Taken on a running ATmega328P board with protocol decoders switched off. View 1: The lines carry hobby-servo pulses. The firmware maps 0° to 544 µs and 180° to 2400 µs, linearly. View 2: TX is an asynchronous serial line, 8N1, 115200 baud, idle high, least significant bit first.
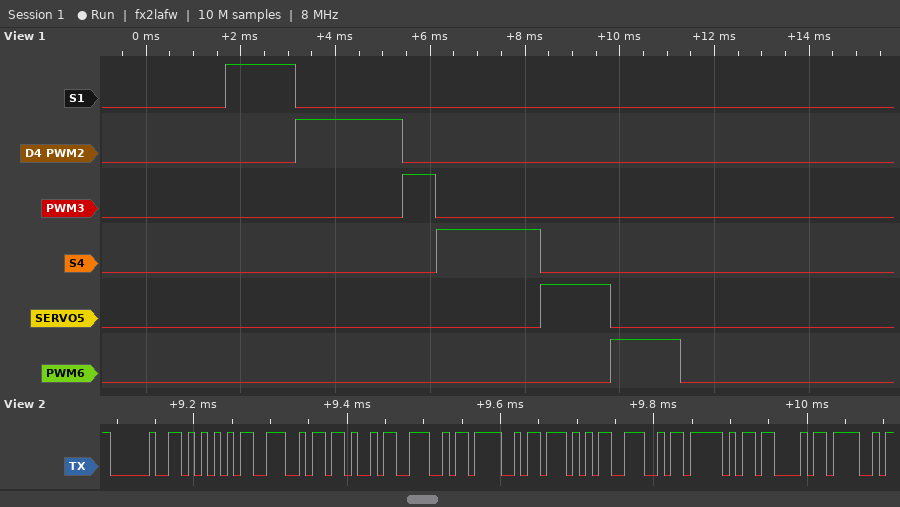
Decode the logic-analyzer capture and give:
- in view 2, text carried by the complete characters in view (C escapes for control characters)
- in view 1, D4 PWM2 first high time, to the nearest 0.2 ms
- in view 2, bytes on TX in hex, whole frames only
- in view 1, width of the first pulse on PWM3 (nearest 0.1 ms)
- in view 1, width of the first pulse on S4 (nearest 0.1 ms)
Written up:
" UNKNOWN_CO"
2.2 ms
0x20 0x55 0x4E 0x4B 0x4E 0x4F 0x57 0x4E 0x5F 0x43 0x4F
0.7 ms
2.2 ms
